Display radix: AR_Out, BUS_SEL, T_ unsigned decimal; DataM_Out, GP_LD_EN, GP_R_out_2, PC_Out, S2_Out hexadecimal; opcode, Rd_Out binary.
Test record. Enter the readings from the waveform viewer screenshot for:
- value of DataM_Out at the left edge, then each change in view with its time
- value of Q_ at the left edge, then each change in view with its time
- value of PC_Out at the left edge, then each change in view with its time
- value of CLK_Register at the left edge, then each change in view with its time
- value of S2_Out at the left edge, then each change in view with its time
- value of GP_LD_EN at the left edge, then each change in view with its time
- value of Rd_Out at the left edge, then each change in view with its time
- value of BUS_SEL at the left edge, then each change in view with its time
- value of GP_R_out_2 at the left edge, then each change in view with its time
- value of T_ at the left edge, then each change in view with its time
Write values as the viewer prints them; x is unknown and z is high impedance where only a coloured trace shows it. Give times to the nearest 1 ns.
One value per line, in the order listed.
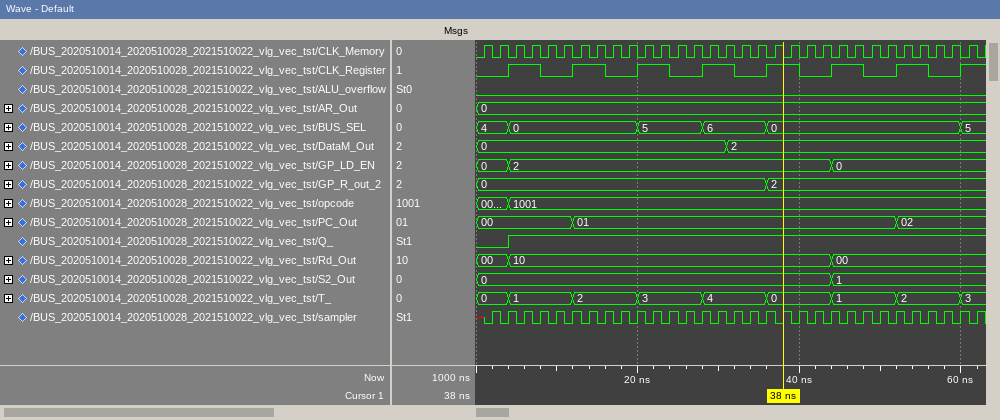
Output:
0, 2 at 31 ns
0, 1 at 4 ns
00, 01 at 12 ns, 02 at 52 ns
0, 1 at 4 ns, 0 at 8 ns, 1 at 12 ns, 0 at 16 ns, 1 at 20 ns, 0 at 24 ns, 1 at 28 ns, 0 at 32 ns, 1 at 36 ns, 0 at 40 ns, 1 at 44 ns, 0 at 48 ns, 1 at 52 ns, 0 at 56 ns, 1 at 60 ns
0, 1 at 44 ns
0, 2 at 4 ns, 0 at 44 ns
00, 10 at 4 ns, 00 at 44 ns
4, 0 at 4 ns, 5 at 20 ns, 6 at 28 ns, 0 at 36 ns, 5 at 60 ns
0, 2 at 36 ns
0, 1 at 4 ns, 2 at 12 ns, 3 at 20 ns, 4 at 28 ns, 0 at 36 ns, 1 at 44 ns, 2 at 52 ns, 3 at 60 ns
